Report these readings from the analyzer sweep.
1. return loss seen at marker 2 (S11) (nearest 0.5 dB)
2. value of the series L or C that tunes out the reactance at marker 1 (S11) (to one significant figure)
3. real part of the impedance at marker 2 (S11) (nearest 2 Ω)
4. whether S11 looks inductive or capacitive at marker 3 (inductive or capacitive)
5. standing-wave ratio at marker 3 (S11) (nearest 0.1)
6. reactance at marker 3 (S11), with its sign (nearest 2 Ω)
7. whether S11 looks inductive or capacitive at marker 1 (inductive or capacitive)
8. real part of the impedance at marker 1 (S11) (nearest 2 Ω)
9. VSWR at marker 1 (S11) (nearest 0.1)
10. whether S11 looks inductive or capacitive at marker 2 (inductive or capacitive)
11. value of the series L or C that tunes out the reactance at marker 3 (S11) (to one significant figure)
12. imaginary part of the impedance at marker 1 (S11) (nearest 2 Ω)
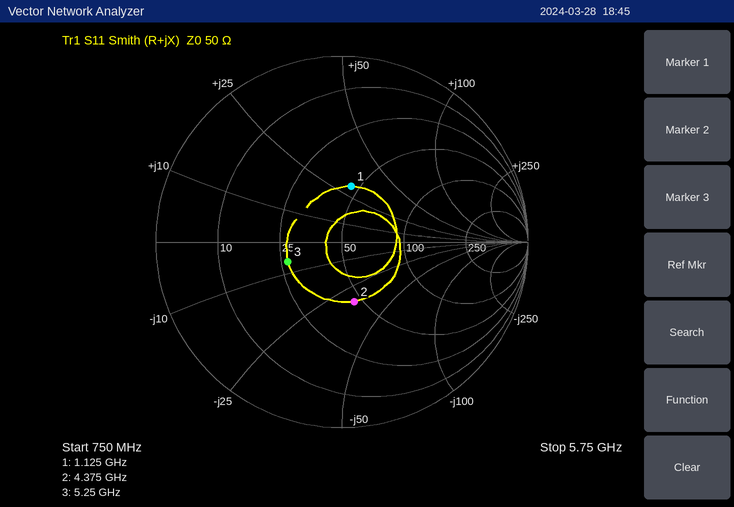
9.5 dB
5 pF
46 Ω
capacitive
1.9
-6 Ω
inductive
46 Ω
1.9
capacitive
200 pH
+30 Ω
